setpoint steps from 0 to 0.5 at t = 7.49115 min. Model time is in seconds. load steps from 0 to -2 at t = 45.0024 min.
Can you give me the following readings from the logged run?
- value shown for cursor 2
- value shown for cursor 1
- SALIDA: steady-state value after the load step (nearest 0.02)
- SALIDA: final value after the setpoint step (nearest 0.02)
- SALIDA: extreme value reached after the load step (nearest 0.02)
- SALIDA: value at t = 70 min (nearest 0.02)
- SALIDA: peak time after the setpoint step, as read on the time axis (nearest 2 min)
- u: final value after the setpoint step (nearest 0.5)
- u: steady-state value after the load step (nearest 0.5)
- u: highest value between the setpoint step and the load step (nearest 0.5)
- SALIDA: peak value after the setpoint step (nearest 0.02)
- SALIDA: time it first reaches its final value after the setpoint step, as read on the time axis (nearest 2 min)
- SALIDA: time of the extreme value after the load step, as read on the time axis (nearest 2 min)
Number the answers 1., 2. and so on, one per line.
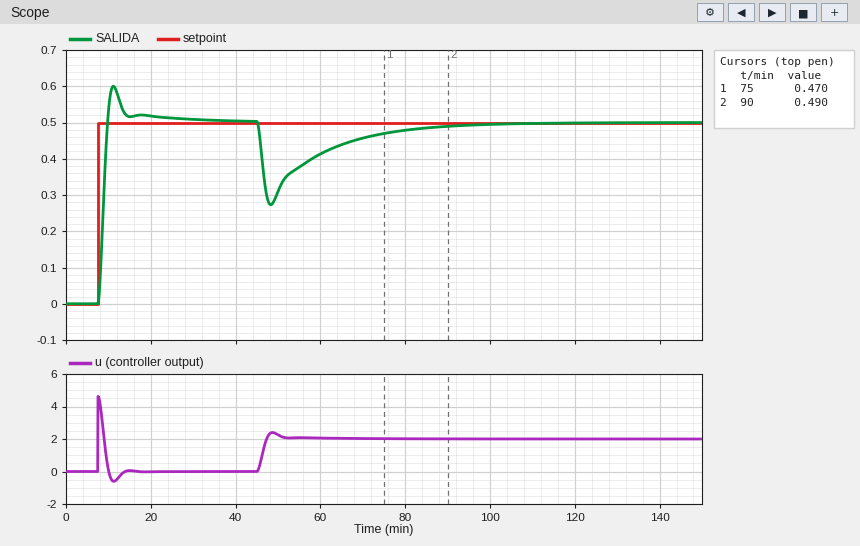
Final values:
1. 0.490
2. 0.470
3. 0.50
4. 0.50
5. 0.28
6. 0.46
7. 12 min
8. 0.0
9. 2.0
10. 4.5
11. 0.60
12. 10 min
13. 48 min
